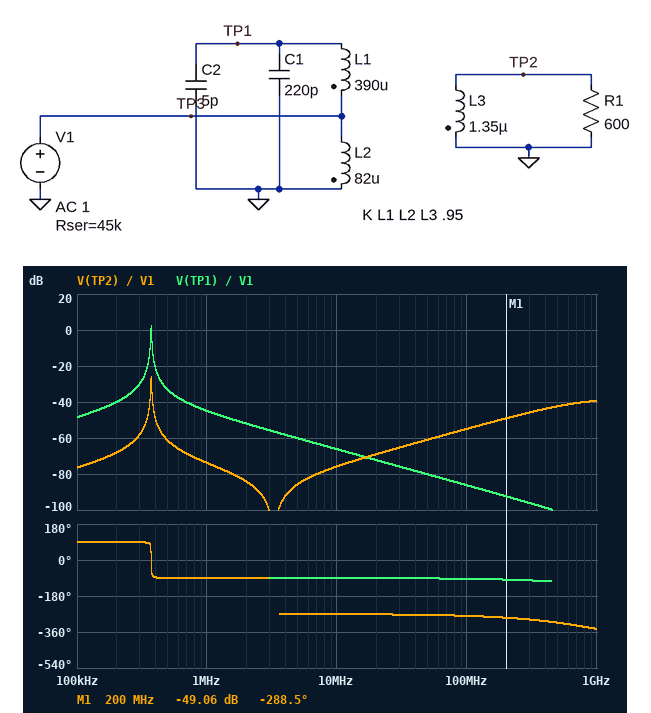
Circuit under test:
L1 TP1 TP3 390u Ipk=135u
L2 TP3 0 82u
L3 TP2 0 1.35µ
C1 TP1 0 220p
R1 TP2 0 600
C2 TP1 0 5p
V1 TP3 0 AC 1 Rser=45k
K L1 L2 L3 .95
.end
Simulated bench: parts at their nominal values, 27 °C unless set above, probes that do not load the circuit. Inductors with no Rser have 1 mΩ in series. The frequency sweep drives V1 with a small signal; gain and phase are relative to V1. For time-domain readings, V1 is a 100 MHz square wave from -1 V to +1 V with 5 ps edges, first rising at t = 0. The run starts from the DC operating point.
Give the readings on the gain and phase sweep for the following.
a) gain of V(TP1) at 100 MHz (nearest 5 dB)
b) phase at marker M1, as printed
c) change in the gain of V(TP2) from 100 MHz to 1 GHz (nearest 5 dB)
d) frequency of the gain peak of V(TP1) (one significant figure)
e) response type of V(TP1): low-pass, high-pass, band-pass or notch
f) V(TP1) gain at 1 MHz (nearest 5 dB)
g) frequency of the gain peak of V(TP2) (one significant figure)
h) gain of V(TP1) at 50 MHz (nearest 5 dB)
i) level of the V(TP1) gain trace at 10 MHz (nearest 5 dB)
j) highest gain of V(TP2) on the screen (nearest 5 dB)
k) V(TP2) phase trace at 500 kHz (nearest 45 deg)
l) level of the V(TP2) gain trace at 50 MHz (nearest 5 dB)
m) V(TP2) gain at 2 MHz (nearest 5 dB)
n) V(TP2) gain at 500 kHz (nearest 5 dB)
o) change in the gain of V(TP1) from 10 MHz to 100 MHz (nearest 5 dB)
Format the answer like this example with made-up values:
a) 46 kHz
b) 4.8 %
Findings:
a) -85 dB
b) -288.5 deg
c) 15 dB
d) 400 kHz
e) band-pass
f) -45 dB
g) 400 kHz
h) -80 dB
i) -65 dB
j) -25 dB
k) -90 deg
l) -60 dB
m) -85 dB
n) -60 dB
o) -20 dB
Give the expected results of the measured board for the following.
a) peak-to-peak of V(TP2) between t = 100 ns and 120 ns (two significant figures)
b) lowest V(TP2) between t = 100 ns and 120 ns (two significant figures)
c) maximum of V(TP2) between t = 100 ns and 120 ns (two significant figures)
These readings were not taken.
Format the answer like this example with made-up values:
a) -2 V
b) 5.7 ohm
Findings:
a) 34 mV
b) -17 mV
c) 17 mV
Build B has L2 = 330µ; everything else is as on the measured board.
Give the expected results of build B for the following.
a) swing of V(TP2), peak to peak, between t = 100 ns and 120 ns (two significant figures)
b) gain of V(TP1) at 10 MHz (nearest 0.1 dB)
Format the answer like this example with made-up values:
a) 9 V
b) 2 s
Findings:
a) 4.0 mV
b) -62.5 dB
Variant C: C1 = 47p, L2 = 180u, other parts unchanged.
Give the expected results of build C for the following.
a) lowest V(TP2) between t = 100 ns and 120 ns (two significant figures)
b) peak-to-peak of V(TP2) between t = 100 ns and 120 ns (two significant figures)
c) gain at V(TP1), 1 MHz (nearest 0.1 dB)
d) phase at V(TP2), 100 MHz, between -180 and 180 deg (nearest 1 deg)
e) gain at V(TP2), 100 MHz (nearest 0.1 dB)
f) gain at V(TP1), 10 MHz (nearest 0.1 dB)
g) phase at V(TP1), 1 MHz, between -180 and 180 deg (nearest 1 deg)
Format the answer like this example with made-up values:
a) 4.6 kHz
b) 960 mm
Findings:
a) -8.5 mV
b) 18 mV
c) -26.0 dB
d) 79 deg
e) -58.5 dB
f) -51.2 dB
g) -88 deg
